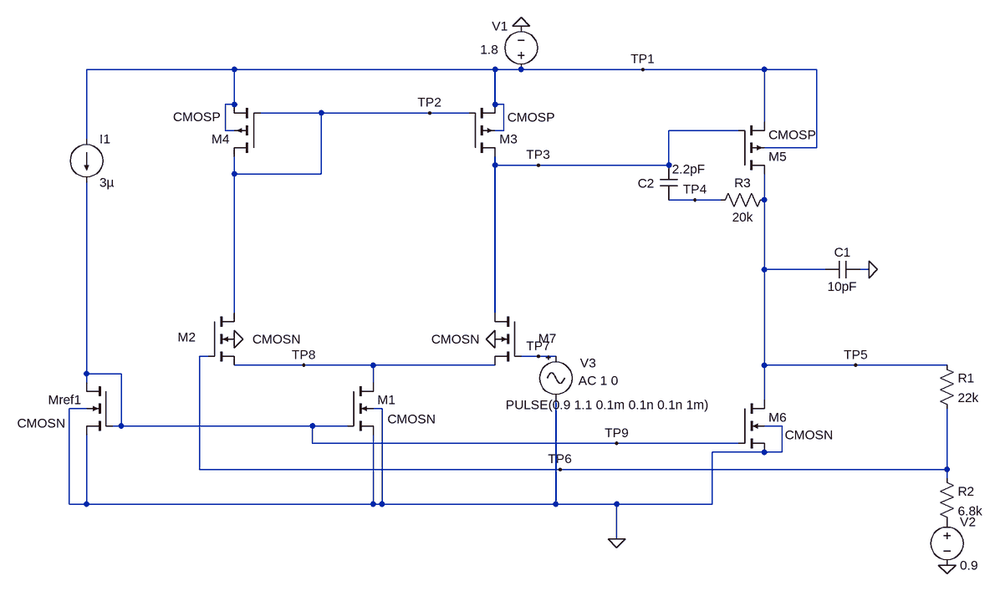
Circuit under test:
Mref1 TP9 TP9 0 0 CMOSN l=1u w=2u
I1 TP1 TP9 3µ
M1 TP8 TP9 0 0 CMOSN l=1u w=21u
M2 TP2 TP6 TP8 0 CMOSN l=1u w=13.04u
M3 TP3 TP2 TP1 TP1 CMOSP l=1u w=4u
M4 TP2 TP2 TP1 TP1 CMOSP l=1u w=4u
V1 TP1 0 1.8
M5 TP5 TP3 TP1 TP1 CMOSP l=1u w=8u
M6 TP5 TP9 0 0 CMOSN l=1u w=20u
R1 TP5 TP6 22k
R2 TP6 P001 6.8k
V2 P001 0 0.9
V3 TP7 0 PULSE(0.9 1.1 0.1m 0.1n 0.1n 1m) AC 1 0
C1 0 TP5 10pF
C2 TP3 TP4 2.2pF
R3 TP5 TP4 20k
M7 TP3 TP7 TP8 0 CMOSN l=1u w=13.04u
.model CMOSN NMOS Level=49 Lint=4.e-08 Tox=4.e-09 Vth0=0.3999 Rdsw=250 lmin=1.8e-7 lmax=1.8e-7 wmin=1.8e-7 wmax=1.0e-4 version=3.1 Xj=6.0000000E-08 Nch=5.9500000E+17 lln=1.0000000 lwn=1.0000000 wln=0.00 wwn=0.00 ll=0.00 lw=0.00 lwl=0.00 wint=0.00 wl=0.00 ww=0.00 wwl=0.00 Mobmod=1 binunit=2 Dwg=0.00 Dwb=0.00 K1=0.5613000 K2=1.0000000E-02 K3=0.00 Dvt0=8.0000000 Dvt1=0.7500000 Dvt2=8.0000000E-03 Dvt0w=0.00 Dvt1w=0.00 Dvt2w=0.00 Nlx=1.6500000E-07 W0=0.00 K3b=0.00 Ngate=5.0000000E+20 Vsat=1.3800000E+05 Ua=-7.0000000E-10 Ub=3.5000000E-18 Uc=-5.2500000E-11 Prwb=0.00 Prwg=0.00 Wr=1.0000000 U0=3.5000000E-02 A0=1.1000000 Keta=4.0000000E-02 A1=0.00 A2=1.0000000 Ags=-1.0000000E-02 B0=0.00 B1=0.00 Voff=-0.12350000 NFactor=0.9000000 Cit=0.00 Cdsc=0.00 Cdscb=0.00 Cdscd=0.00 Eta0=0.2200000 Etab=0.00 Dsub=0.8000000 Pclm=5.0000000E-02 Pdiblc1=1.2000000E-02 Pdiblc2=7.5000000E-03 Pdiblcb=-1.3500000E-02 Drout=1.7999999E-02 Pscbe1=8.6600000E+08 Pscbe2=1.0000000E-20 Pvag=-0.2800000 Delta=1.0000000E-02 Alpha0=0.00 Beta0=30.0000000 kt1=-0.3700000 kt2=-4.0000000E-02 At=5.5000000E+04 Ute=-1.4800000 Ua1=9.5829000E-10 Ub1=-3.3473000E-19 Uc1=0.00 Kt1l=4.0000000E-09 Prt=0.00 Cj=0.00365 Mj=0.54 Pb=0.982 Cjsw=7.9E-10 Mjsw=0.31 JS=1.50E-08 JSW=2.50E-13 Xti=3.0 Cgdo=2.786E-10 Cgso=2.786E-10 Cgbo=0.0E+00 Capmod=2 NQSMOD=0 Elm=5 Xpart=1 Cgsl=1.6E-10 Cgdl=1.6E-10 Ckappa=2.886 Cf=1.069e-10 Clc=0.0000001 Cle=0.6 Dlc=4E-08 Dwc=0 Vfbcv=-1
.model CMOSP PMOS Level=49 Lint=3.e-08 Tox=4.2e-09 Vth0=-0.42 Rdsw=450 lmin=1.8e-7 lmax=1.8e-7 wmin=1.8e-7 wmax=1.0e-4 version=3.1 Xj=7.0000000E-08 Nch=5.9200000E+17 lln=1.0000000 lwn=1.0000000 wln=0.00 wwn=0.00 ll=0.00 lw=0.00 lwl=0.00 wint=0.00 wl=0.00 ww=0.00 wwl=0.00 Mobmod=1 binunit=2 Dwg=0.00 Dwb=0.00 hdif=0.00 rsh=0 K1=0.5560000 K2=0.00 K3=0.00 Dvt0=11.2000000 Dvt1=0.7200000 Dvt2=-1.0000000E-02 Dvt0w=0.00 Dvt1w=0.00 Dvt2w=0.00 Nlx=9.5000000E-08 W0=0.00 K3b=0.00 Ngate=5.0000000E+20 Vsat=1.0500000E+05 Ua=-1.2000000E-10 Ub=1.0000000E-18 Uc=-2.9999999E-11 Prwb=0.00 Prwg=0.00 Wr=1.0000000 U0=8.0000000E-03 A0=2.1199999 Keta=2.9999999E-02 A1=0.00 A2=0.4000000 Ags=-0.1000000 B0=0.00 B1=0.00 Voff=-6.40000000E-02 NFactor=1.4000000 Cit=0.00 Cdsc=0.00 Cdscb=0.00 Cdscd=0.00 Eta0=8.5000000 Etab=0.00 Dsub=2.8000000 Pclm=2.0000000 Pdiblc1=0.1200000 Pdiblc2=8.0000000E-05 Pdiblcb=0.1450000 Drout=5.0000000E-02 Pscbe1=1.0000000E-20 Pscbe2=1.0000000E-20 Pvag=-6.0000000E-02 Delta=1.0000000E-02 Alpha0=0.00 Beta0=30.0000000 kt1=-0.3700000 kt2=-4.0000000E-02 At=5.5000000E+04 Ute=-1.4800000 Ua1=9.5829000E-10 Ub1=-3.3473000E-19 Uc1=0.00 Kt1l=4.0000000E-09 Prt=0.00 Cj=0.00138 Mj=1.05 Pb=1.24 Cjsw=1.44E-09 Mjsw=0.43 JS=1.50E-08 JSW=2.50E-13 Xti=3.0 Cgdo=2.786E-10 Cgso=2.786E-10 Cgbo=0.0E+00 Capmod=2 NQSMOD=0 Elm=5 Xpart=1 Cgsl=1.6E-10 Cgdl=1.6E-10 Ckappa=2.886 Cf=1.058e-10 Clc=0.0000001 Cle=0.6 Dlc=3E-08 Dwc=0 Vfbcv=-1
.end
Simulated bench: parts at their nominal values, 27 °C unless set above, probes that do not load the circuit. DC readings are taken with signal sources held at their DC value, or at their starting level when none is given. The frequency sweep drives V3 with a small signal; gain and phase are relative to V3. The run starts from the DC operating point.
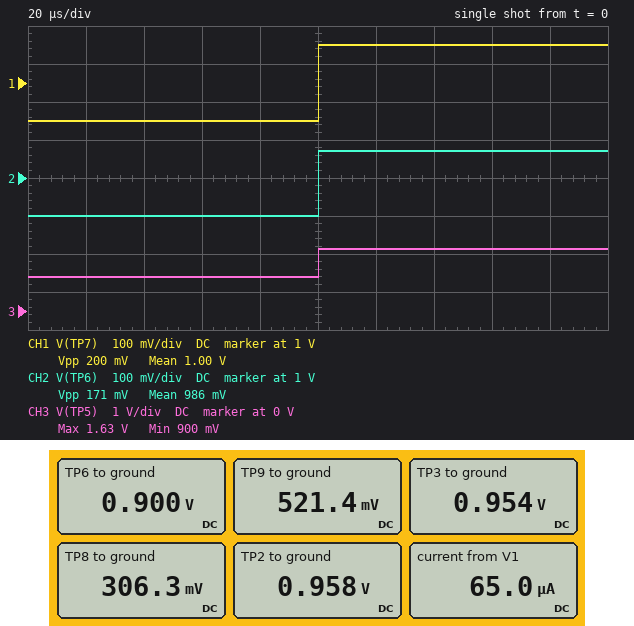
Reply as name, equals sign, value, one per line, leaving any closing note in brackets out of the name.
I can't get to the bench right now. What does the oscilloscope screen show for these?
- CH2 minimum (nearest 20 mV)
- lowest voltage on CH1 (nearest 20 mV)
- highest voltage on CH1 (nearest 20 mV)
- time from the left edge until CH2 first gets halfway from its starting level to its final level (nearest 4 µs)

CH2 minimum = 900 mV
lowest voltage on CH1 = 900 mV
highest voltage on CH1 = 1.10 V
time from the left edge until CH2 first gets halfway from its starting level to its final level = 100 µs
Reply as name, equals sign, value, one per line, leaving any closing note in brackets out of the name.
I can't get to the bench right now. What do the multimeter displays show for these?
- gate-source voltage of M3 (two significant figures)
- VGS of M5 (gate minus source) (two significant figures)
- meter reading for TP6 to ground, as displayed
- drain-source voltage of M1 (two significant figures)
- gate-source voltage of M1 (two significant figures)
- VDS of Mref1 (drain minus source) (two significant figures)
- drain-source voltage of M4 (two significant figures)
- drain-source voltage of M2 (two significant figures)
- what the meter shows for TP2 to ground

gate-source voltage of M3 = -840 mV
VGS of M5 (gate minus source) = -850 mV
meter reading for TP6 to ground, as displayed = 0.900 V
drain-source voltage of M1 = 310 mV
gate-source voltage of M1 = 520 mV
VDS of Mref1 (drain minus source) = 520 mV
drain-source voltage of M4 = -840 mV
drain-source voltage of M2 = 650 mV
what the meter shows for TP2 to ground = 0.958 V
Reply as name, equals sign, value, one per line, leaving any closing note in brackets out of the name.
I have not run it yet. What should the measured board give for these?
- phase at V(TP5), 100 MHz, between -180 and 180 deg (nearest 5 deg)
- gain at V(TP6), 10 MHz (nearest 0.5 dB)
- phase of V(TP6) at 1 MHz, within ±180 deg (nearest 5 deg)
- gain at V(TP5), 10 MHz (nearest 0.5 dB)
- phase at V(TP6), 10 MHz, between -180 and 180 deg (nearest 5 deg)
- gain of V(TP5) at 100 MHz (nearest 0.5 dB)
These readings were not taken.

phase at V(TP5), 100 MHz, between -180 and 180 deg = -160 deg
gain at V(TP6), 10 MHz = -16.0 dB
phase of V(TP6) at 1 MHz, within ±180 deg = -20 deg
gain at V(TP5), 10 MHz = -3.0 dB
phase at V(TP6), 10 MHz, between -180 and 180 deg = -105 deg
gain of V(TP5) at 100 MHz = -28.5 dB
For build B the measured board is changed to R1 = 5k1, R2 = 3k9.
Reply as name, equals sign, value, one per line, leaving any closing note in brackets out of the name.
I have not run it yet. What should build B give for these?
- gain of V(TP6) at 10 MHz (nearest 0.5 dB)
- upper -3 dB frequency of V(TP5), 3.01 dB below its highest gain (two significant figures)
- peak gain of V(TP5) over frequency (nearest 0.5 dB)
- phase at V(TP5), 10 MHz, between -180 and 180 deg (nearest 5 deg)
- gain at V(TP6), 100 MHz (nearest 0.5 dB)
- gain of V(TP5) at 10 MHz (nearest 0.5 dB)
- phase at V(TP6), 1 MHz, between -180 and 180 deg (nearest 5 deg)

gain of V(TP6) at 10 MHz = -11.0 dB
upper -3 dB frequency of V(TP5), 3.01 dB below its highest gain = 4.0 MHz
peak gain of V(TP5) over frequency = 7.0 dB
phase at V(TP5), 10 MHz, between -180 and 180 deg = -90 deg
gain at V(TP6), 100 MHz = -27.5 dB
gain of V(TP5) at 10 MHz = -3.5 dB
phase at V(TP6), 1 MHz, between -180 and 180 deg = -15 deg
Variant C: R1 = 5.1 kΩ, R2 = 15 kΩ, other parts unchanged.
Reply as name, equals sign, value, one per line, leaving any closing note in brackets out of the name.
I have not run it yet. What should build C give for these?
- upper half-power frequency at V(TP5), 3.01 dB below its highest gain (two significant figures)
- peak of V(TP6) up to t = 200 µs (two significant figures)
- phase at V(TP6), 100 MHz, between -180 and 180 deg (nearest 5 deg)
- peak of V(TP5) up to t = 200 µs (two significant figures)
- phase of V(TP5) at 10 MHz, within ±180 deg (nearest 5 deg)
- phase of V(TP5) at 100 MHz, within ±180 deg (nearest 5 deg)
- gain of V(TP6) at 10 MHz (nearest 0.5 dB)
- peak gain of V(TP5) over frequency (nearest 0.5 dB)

upper half-power frequency at V(TP5), 3.01 dB below its highest gain = 7.1 MHz
peak of V(TP6) up to t = 200 µs = 1.1 V
phase at V(TP6), 100 MHz, between -180 and 180 deg = 90 deg
peak of V(TP5) up to t = 200 µs = 1.2 V
phase of V(TP5) at 10 MHz, within ±180 deg = -80 deg
phase of V(TP5) at 100 MHz, within ±180 deg = -155 deg
gain of V(TP6) at 10 MHz = -6.0 dB
peak gain of V(TP5) over frequency = 3.0 dB
